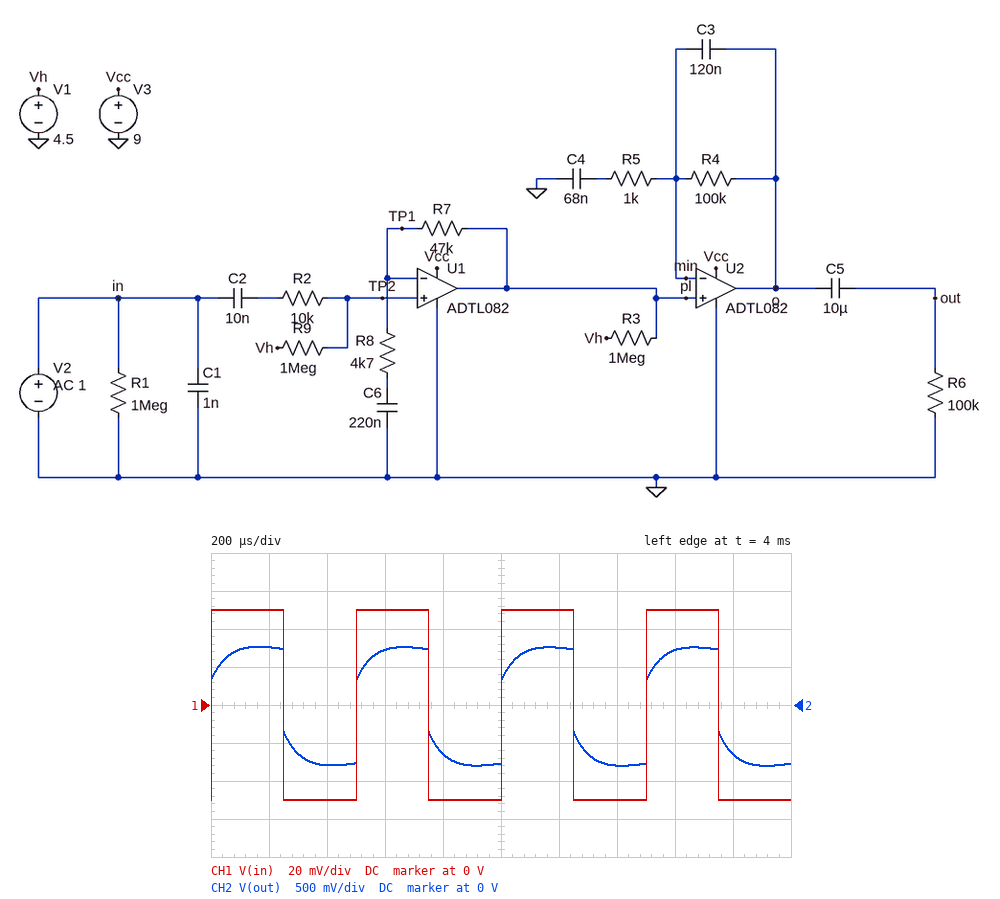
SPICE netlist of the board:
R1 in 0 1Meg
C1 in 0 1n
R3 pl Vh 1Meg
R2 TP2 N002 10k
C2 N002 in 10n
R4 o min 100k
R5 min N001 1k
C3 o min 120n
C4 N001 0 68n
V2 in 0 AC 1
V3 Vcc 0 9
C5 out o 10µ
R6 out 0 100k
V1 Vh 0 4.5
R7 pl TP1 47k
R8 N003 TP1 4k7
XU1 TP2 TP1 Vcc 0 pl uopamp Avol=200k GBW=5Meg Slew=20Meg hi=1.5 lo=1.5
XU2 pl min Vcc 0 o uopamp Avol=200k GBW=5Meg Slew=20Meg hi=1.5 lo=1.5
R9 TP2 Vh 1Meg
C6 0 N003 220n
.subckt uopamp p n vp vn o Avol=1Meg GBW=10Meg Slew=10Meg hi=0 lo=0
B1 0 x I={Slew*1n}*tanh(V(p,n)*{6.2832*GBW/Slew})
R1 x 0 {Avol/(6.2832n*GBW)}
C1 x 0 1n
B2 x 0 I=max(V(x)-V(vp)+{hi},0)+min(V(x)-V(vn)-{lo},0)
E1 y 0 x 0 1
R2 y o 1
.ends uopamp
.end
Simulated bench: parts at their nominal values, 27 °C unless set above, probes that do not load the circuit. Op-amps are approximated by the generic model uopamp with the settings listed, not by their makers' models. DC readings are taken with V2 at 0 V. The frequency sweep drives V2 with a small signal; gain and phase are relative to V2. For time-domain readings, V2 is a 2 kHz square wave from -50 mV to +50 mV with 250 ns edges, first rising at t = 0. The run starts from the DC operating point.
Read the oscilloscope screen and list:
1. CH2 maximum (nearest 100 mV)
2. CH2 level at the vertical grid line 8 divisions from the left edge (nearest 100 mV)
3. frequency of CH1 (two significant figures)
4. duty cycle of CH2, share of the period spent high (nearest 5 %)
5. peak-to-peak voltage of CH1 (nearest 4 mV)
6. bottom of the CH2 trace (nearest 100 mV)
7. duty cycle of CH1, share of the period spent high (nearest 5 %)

800 mV
700 mV
2.0 kHz
50 %
100 mV
-800 mV
50 %
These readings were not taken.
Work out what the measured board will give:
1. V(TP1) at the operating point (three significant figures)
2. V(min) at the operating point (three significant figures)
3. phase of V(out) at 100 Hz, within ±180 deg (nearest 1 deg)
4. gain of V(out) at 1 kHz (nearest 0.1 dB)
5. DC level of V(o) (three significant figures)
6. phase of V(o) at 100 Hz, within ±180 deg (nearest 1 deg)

4.50 V
4.50 V
60 deg
24.1 dB
4.50 V
60 deg
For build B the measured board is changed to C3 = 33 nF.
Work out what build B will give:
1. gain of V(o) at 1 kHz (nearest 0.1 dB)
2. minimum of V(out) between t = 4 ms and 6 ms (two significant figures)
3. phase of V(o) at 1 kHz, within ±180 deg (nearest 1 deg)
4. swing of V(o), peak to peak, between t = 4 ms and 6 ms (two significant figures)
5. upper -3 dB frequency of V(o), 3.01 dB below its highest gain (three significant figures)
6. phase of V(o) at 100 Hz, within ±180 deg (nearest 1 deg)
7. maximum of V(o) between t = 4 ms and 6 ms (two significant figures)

29.7 dB
-1.6 V
-5 deg
3.0 V
3.01 kHz
73 deg
5.9 V
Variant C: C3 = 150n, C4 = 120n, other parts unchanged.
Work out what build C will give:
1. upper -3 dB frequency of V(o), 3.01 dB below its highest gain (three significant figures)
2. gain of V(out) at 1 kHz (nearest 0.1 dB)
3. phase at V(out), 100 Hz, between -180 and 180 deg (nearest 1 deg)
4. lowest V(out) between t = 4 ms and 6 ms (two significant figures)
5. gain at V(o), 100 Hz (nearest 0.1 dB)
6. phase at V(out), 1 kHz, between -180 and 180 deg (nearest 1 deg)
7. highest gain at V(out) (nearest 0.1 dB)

3.04 kHz
24.5 dB
59 deg
-830 mV
20.5 dB
-5 deg
25.1 dB
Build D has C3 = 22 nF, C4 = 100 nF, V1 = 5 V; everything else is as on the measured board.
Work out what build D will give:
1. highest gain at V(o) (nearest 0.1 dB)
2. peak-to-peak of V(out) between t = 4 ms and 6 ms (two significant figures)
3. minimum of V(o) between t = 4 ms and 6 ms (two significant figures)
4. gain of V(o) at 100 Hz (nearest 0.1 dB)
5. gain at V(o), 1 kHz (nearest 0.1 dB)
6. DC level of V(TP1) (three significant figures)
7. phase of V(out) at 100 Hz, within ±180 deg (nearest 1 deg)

34.8 dB
4.9 V
2.4 V
28.6 dB
34.2 dB
5.00 V
84 deg
